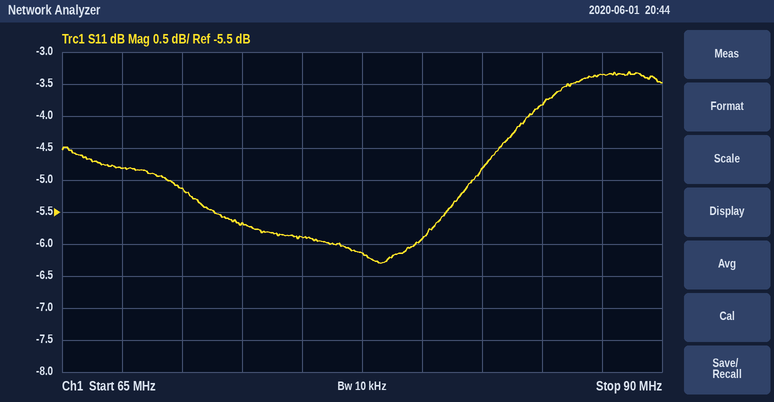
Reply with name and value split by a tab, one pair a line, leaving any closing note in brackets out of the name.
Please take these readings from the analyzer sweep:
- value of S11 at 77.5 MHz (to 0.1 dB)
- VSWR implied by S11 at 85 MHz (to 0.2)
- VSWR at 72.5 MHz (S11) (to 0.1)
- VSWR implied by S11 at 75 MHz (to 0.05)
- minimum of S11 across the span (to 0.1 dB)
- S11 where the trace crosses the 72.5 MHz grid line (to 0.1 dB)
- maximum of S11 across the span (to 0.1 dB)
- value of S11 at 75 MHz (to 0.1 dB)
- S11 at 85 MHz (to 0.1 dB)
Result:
value of S11 at 77.5 MHz	-6.1 dB
VSWR implied by S11 at 85 MHz	4.6
VSWR at 72.5 MHz (S11)	3.2
VSWR implied by S11 at 75 MHz	3.05
minimum of S11 across the span	-6.3 dB
S11 where the trace crosses the 72.5 MHz grid line	-5.7 dB
maximum of S11 across the span	-3.3 dB
value of S11 at 75 MHz	-5.9 dB
S11 at 85 MHz	-3.8 dB
